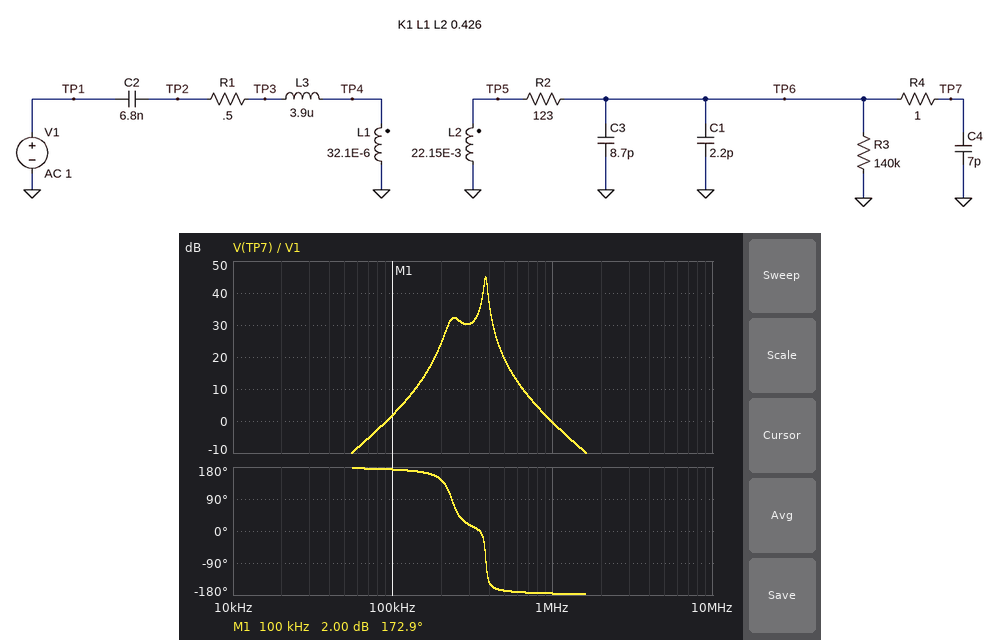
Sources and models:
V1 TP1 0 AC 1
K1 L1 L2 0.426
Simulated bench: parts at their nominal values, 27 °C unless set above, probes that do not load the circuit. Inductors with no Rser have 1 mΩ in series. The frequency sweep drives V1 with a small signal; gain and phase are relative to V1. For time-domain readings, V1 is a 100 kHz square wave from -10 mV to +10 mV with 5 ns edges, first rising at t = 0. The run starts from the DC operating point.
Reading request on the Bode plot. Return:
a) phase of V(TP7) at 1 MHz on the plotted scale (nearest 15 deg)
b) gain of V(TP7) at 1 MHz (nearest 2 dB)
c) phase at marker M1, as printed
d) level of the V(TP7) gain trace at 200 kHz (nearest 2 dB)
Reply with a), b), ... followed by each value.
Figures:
a) -180 deg
b) 0 dB
c) 172.9 deg
d) 24 dB
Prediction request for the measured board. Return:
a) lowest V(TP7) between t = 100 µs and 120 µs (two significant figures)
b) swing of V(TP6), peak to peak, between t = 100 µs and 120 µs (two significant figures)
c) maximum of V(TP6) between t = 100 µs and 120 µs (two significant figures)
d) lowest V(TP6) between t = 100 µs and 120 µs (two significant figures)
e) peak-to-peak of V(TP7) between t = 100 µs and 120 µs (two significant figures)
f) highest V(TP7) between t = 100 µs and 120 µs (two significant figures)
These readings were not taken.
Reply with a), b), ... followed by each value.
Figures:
a) -170 mV
b) 350 mV
c) 170 mV
d) -170 mV
e) 350 mV
f) 170 mV
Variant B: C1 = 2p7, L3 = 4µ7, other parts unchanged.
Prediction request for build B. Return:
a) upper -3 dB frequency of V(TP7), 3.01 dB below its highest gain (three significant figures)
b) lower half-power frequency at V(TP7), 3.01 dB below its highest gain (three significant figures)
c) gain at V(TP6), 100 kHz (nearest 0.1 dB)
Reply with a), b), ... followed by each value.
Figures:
a) 382 kHz
b) 365 kHz
c) 2.1 dB
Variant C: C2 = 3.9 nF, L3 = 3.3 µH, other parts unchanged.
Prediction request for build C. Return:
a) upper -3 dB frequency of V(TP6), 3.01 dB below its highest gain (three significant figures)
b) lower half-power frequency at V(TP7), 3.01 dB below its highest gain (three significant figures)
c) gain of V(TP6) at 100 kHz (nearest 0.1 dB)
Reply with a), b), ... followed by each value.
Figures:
a) 491 kHz
b) 482 kHz
c) -3.2 dB
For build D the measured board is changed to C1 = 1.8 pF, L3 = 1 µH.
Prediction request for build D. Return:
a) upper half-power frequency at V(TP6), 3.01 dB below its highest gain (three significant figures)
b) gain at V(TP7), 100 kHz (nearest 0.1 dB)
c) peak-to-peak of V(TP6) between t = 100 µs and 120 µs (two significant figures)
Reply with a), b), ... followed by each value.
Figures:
a) 407 kHz
b) 1.9 dB
c) 340 mV
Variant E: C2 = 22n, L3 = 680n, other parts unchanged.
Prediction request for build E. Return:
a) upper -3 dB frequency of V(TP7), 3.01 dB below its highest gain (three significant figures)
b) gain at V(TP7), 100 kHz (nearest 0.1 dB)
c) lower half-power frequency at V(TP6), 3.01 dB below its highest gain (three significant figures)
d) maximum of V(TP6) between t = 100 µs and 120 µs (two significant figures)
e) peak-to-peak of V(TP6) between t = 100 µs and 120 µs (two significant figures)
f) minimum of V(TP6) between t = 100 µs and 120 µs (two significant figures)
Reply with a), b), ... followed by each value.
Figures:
a) 184 kHz
b) 14.3 dB
c) 169 kHz
d) 400 mV
e) 790 mV
f) -400 mV
